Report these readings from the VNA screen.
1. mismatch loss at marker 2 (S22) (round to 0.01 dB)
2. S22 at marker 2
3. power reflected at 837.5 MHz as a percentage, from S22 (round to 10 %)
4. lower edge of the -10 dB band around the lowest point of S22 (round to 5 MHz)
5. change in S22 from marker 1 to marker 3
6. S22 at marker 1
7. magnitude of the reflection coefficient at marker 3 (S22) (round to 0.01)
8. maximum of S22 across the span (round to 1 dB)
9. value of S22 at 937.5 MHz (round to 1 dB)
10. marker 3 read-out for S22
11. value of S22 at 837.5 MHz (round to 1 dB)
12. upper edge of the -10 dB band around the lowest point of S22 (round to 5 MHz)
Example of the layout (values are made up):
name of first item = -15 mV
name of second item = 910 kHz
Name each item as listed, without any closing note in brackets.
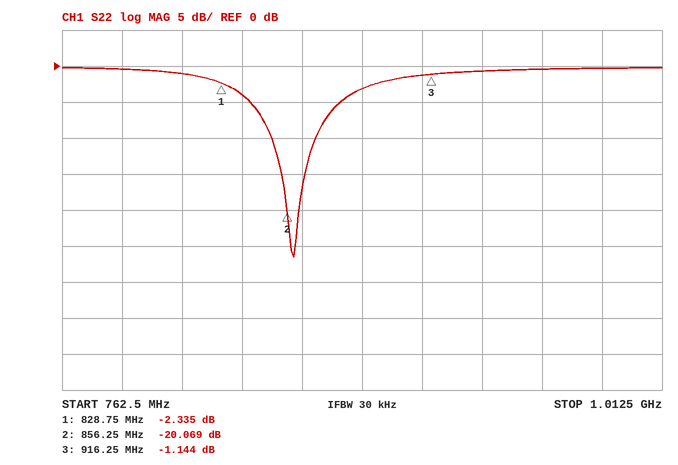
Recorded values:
mismatch loss at marker 2 (S22) = 0.04 dB
S22 at marker 2 = -20.069 dB
power reflected at 837.5 MHz as a percentage, from S22 = 40 %
lower edge of the -10 dB band around the lowest point of S22 = 850 MHz
change in S22 from marker 1 to marker 3 = 1.191 dB
S22 at marker 1 = -2.335 dB
magnitude of the reflection coefficient at marker 3 (S22) = 0.88
maximum of S22 across the span = 0 dB
value of S22 at 937.5 MHz = -1 dB
marker 3 read-out for S22 = -1.144 dB
value of S22 at 837.5 MHz = -4 dB
upper edge of the -10 dB band around the lowest point of S22 = 870 MHz
